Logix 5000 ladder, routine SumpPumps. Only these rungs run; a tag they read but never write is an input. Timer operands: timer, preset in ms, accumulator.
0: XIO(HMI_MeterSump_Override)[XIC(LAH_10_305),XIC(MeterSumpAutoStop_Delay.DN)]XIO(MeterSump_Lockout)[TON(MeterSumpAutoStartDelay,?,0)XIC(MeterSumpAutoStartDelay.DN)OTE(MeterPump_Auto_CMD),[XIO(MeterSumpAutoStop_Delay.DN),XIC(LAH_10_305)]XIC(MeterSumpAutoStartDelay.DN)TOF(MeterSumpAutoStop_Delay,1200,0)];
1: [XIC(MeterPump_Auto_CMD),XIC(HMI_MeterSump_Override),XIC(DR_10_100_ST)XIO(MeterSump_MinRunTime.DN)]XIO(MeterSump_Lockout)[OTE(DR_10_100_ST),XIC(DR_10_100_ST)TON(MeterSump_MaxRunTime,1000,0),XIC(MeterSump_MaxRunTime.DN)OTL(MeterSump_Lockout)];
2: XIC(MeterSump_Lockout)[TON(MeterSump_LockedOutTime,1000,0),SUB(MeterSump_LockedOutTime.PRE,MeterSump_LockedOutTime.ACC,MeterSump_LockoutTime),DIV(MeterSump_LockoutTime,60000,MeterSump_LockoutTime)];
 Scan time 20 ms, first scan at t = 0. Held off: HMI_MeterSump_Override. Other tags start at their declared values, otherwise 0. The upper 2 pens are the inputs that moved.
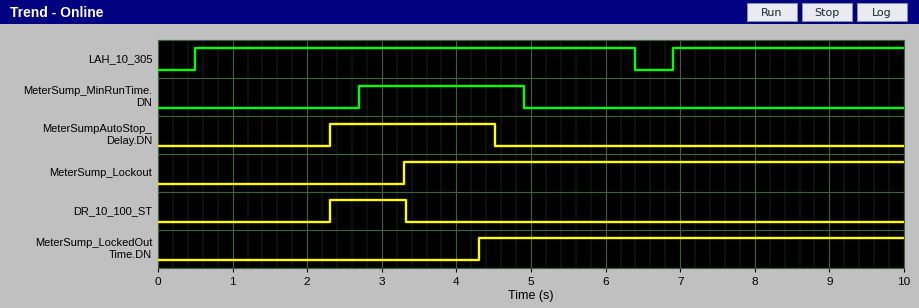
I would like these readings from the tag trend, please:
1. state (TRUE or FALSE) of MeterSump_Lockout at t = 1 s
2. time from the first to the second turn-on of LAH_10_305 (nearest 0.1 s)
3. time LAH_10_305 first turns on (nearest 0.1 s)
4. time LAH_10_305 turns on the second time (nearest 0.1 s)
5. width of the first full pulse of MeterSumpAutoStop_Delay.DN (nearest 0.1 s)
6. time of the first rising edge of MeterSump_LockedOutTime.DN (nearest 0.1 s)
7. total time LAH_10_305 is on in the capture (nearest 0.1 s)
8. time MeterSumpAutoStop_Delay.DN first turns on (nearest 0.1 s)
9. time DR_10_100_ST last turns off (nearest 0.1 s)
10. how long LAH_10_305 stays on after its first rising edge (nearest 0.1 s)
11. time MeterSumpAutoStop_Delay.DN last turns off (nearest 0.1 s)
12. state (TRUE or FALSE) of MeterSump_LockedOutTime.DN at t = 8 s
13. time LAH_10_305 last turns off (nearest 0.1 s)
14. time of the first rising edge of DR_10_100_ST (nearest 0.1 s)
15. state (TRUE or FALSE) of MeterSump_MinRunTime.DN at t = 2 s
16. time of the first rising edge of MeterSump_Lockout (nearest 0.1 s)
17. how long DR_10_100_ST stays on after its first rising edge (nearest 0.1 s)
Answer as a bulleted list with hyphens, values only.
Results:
- FALSE
- 6.4 s
- 0.5 s
- 6.9 s
- 2.2 s
- 4.3 s
- 9.0 s
- 2.3 s
- 3.3 s
- 5.9 s
- 4.5 s
- TRUE
- 6.4 s
- 2.3 s
- FALSE
- 3.3 s
- 1.0 s
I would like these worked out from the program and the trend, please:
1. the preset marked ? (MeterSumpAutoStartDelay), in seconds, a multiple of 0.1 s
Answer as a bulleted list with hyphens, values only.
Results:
- 1.8 s
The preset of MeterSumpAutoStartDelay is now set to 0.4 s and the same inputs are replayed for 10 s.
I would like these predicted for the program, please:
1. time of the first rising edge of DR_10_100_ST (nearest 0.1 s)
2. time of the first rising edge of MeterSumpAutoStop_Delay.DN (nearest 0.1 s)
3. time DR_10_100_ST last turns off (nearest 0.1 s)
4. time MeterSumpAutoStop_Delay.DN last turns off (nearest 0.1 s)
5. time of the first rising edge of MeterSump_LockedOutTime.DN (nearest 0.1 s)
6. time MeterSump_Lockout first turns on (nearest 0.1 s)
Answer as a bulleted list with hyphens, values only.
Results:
- 0.9 s
- 0.9 s
- 1.9 s
- 3.1 s
- 2.9 s
- 1.9 s
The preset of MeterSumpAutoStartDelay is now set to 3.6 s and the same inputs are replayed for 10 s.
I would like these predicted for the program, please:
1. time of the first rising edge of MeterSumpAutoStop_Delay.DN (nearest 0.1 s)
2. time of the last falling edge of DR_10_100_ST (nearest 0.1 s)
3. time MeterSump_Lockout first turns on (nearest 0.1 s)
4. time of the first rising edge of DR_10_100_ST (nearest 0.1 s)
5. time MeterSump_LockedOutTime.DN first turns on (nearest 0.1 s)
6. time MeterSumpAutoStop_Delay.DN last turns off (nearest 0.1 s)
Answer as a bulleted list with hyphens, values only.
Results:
- 4.1 s
- 5.1 s
- 5.1 s
- 4.1 s
- 6.1 s
- 6.3 s
